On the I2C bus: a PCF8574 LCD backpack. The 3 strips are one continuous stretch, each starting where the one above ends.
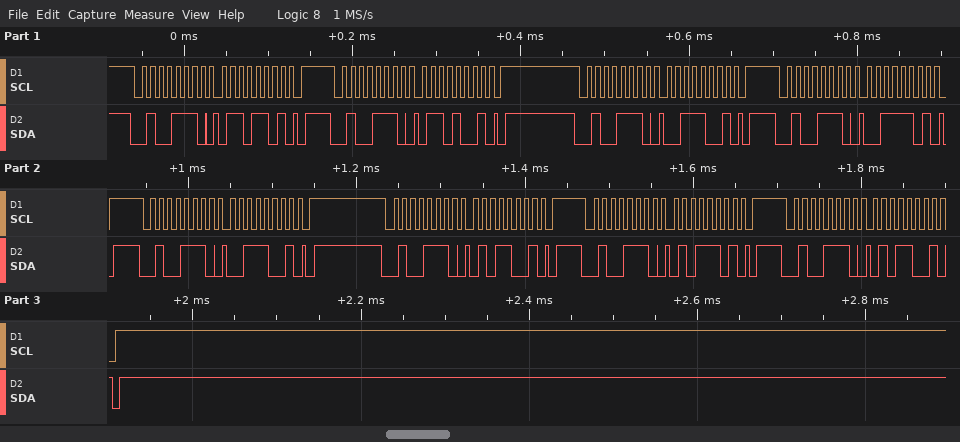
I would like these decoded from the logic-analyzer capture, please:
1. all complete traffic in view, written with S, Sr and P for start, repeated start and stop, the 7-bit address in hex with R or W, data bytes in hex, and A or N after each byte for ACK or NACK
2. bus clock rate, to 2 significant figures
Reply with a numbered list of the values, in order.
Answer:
1. S 27W A 6D A P S 27W A 69 A P S 27W A 39 A P S 27W A 3D A P S 27W A 39 A P S 27W A 59 A P S 27W A 5D A P S 27W A 59 A P
2. 100 kHz
